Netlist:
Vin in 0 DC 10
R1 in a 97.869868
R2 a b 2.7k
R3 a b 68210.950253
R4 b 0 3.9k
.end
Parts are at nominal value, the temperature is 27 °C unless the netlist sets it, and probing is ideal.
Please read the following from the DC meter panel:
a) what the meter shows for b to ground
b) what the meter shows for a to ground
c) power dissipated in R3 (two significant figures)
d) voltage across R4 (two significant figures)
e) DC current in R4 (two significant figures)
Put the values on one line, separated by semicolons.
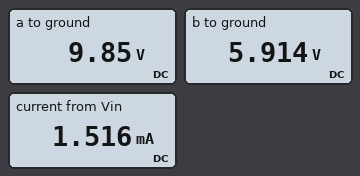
5.914 V; 9.85 V; 230 µW; 5.9 V; 1.5 mA
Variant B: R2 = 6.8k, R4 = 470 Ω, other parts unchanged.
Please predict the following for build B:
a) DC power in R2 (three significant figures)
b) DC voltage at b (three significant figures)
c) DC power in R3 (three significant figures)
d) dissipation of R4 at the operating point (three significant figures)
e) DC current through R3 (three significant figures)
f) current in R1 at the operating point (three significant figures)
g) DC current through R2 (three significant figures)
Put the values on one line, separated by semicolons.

12.3 mW; 696 mV; 1.23 mW; 1.03 mW; 134 µA; 1.48 mA; 1.35 mA
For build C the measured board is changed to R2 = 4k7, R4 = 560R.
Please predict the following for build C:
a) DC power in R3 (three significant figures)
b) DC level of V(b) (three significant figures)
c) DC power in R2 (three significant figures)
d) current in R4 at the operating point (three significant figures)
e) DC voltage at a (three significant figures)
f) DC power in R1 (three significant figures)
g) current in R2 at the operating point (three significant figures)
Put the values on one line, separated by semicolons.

1.11 mW; 1.11 V; 16.1 mW; 1.98 mA; 9.81 V; 383 µW; 1.85 mA
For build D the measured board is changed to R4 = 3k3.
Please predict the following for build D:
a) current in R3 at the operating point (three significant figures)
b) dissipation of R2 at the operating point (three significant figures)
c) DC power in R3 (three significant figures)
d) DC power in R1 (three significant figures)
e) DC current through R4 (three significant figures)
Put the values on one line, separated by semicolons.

63.5 µA; 6.95 mW; 275 µW; 272 µW; 1.67 mA
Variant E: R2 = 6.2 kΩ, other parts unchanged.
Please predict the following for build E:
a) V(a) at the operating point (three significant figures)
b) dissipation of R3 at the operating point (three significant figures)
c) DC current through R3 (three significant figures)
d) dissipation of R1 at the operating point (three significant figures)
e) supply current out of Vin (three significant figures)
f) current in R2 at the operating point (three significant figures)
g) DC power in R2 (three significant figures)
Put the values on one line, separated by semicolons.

9.90 V; 505 µW; 86.1 µA; 104 µW; 1.03 mA; 947 µA; 5.56 mW
